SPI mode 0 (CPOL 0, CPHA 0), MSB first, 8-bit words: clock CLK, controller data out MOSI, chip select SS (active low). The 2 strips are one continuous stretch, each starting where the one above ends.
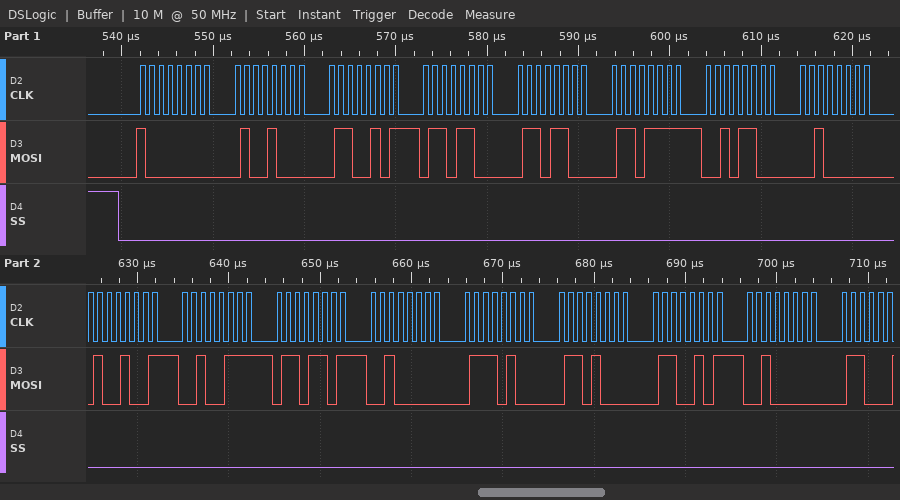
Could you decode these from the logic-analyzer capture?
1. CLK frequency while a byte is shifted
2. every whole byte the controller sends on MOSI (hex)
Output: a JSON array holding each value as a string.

["1 MHz", "80 48 65 6C 6C 6F 2C 20 49 27 6D 20 74 68 65 20"]
